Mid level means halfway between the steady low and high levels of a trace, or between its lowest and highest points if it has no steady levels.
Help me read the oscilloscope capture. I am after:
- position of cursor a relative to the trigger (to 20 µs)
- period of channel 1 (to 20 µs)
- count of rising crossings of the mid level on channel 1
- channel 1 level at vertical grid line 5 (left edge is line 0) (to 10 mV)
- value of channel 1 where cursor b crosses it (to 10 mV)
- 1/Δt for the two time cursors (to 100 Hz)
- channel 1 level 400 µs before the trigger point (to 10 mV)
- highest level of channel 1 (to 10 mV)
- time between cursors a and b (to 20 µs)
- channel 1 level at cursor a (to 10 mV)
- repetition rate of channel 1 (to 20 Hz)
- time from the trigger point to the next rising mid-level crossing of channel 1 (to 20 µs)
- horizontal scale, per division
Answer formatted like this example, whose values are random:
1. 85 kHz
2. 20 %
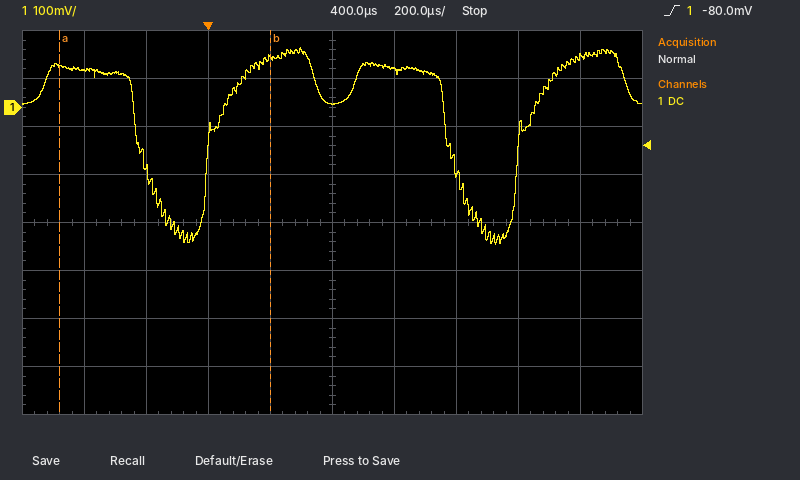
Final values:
1. -480 µs
2. 1.00 ms
3. 2
4. 10 mV
5. 100 mV
6. 1.5 kHz
7. 80 mV
8. 120 mV
9. 680 µs
10. 90 mV
11. 1.00 kHz
12. 1.00 ms
13. 200 µs
